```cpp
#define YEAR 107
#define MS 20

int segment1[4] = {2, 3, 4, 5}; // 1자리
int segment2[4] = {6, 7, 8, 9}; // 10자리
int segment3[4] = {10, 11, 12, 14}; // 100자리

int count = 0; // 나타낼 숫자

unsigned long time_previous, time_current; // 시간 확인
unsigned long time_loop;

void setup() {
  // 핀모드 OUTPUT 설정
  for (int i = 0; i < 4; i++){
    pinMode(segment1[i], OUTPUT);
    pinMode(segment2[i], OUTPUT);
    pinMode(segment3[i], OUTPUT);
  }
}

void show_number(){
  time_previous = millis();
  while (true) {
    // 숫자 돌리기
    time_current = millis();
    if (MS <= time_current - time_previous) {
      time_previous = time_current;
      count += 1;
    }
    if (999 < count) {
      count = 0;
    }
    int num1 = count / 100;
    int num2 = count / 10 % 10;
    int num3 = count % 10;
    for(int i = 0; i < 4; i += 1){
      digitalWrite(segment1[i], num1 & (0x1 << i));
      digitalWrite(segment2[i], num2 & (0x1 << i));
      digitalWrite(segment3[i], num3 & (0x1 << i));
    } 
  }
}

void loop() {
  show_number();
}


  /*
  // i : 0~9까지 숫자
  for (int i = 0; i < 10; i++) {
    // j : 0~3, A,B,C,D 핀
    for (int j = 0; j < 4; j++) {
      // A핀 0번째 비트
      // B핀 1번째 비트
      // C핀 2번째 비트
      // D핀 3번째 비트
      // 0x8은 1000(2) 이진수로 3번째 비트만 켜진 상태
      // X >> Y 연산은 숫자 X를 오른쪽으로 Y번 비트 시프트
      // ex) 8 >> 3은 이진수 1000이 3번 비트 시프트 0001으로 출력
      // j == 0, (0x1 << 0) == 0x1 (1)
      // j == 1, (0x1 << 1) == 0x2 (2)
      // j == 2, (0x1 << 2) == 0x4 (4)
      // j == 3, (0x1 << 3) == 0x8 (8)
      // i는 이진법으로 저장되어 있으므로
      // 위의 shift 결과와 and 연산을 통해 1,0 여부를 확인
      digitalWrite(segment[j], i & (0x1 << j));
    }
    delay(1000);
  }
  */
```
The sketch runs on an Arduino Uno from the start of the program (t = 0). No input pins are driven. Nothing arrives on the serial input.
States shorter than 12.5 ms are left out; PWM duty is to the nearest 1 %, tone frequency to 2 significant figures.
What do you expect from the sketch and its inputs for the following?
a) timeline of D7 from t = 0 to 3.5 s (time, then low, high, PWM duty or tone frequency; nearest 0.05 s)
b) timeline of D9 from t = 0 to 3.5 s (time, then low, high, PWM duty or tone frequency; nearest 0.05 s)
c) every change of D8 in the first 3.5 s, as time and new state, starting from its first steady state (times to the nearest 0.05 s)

0 s low; 0.4 s high; 0.8 s low; 1.2 s high; 1.6 s low; 2.4 s high; 2.8 s low; 3.2 s high
0 s low; 1.6 s high; 2 s low
0 s low; 0.8 s high; 1.6 s low; 2.8 s high
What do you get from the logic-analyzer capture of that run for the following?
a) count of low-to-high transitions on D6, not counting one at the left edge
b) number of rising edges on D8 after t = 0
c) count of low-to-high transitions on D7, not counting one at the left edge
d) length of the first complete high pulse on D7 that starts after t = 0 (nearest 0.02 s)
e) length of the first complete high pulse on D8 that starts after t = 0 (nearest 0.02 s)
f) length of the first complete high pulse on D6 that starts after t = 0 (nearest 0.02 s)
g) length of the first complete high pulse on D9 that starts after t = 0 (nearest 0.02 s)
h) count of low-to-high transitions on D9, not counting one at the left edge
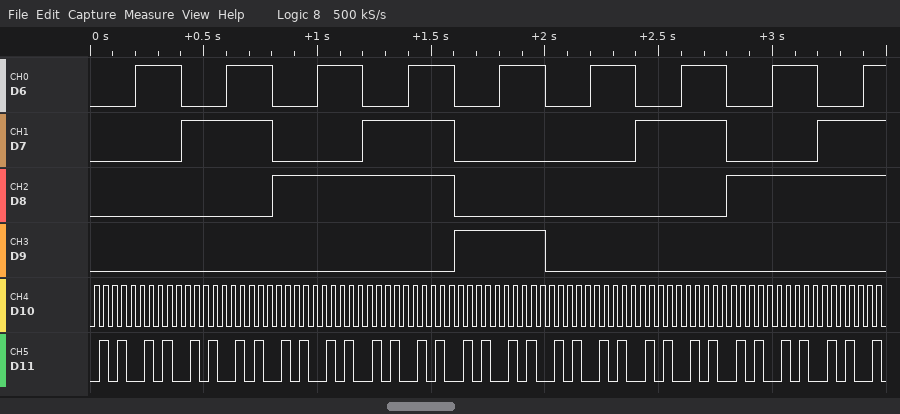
9
2
4
0.40 s
0.80 s
0.20 s
0.40 s
1
